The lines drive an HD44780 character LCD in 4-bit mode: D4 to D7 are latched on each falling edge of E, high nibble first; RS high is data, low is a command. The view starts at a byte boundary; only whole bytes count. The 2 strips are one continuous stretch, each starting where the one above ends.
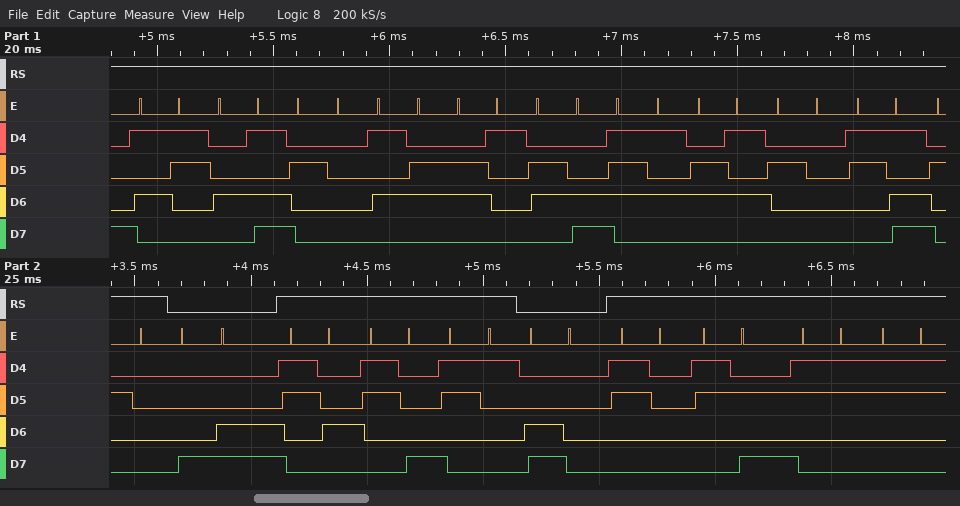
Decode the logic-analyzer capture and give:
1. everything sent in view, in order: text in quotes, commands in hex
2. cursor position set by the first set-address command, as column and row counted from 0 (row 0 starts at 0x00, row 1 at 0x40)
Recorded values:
"SM Value = " 0x8C "481" 0xC0 "0:33"
column 12, row 0
